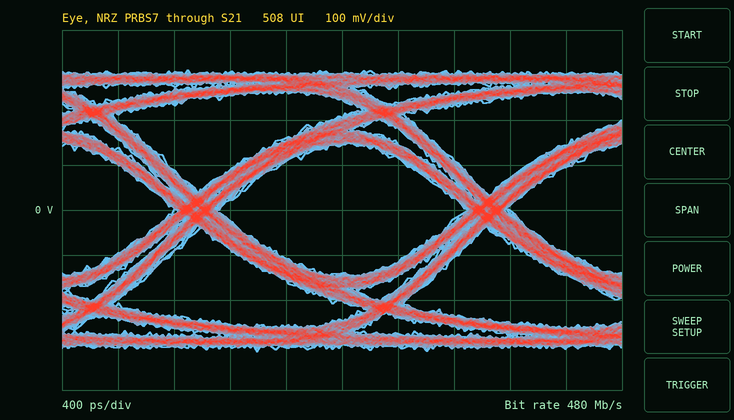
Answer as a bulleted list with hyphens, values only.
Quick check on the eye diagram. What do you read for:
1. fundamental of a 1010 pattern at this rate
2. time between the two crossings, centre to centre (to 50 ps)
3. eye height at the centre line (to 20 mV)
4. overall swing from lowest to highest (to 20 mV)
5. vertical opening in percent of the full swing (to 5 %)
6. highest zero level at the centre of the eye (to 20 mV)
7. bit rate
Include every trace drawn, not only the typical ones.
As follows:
- 240 MHz
- 2.10 ns
- 280 mV
- 620 mV
- 45 %
- -140 mV
- 480 Mb/s
